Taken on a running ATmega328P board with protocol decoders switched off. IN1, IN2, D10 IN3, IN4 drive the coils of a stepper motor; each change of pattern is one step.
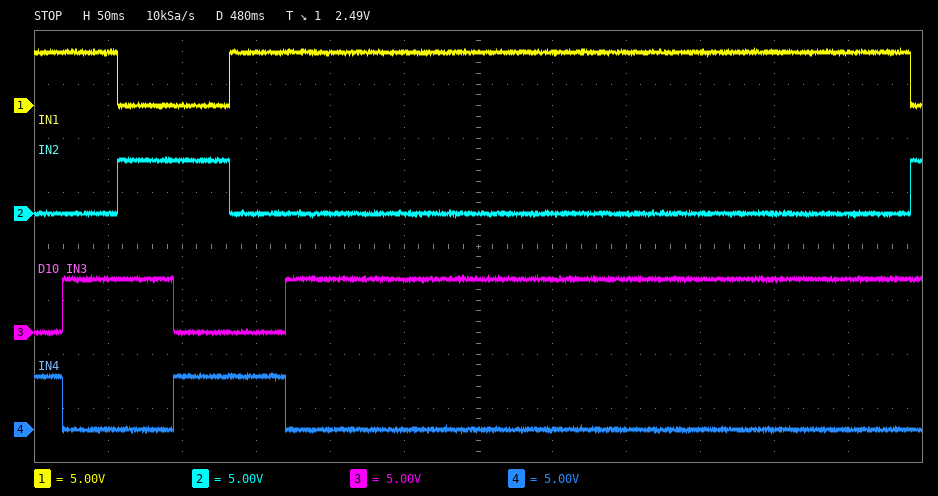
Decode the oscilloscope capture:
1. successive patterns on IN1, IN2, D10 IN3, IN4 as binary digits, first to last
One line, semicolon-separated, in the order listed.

1001 1010 0110 0101 1001 1010 0110
